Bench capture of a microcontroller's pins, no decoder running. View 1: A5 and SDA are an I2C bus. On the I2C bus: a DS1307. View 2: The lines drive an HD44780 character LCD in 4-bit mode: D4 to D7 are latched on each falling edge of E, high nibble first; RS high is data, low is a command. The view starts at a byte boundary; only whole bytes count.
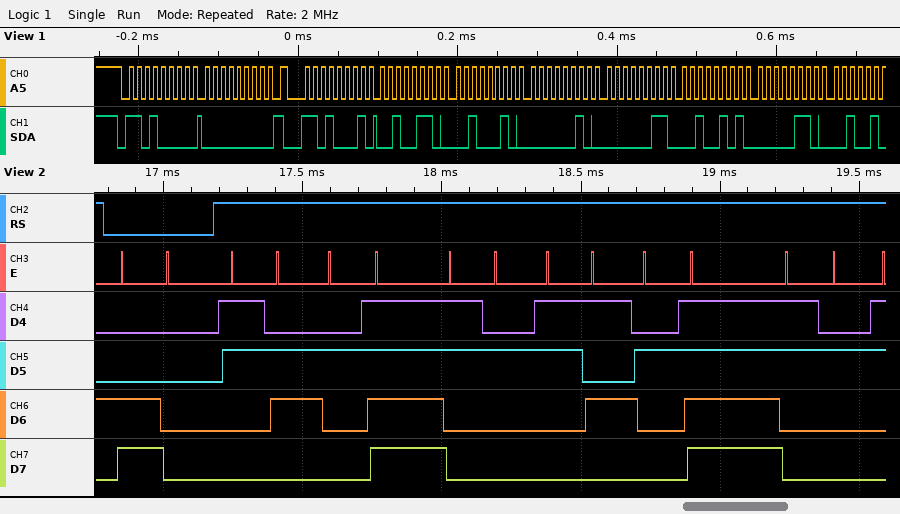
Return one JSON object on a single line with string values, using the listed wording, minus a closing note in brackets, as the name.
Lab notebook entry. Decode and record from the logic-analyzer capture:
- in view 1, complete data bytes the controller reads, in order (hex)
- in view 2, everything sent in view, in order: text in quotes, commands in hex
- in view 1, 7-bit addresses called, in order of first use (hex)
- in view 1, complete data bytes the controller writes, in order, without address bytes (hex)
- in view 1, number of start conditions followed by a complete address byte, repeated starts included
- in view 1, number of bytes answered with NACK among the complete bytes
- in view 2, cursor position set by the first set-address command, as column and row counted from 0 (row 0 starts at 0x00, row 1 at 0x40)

{"in view 1, complete data bytes the controller reads, in order": "26 22 02 03 25 06", "in view 2, everything sent in view, in order: text in quotes, commands in hex": "0xC0 \"6/25/2\"", "in view 1, 7-bit addresses called, in order of first use": "0x68", "in view 1, complete data bytes the controller writes, in order, without address bytes": "00", "in view 1, number of start conditions followed by a complete address byte, repeated starts included": "2", "in view 1, number of bytes answered with NACK among the complete bytes": "0", "in view 2, cursor position set by the first set-address command, as column and row counted from 0": "column 0, row 1"}
